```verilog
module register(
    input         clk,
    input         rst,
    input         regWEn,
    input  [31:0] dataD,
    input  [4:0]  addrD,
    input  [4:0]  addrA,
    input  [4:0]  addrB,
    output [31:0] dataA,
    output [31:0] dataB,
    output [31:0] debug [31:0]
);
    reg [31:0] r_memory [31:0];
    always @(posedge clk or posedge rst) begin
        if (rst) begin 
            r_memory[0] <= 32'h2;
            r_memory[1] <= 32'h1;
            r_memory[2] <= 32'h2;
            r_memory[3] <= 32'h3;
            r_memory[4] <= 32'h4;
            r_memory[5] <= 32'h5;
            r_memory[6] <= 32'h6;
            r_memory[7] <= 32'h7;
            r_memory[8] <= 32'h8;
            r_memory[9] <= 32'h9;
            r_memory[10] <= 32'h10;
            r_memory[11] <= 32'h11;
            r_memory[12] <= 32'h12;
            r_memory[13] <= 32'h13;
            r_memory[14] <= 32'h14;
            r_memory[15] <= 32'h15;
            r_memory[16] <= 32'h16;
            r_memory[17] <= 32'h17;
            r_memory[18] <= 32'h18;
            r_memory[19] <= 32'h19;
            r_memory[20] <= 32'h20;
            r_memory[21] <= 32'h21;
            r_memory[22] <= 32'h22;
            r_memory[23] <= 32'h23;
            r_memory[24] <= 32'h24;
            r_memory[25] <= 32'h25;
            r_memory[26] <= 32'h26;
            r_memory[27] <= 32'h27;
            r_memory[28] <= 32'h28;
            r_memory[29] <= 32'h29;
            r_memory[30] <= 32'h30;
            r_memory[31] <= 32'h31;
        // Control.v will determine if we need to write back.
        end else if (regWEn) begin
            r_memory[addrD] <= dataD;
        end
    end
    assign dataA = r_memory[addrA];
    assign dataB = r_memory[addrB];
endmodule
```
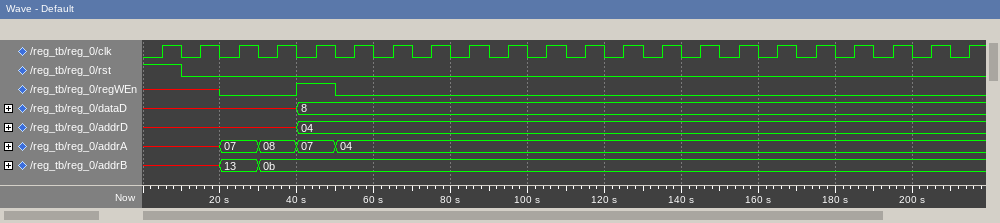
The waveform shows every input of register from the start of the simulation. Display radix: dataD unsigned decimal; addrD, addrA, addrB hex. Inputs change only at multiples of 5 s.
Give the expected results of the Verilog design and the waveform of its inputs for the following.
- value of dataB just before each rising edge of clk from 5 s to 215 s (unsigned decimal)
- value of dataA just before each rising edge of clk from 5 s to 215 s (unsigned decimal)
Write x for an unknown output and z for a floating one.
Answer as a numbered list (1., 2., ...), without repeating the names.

1. x, x, 25, 17, 17, 17, 17, 17, 17, 17, 17, 17, 17, 17, 17, 17, 17, 17, 17, 17, 17, 17
2. x, x, 7, 8, 7, 8, 8, 8, 8, 8, 8, 8, 8, 8, 8, 8, 8, 8, 8, 8, 8, 8
